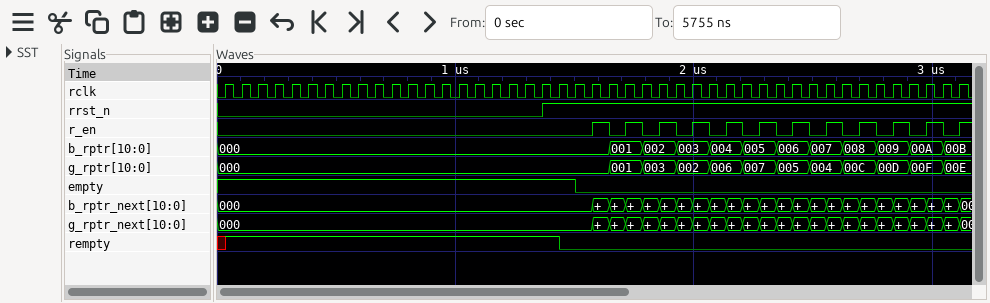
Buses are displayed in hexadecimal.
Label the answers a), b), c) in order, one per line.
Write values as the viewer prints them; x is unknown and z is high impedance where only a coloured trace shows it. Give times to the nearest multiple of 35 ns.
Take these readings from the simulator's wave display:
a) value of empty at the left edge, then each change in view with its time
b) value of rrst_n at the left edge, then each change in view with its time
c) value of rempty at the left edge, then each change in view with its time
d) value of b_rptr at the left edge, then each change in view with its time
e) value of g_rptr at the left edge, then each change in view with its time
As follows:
a) 1, 0 at 1505 ns
b) 0, 1 at 1365 ns
c) x, 1 at 35 ns, 0 at 1435 ns
d) 000, 001 at 1645 ns, 002 at 1785 ns, 003 at 1925 ns, 004 at 2065 ns, 005 at 2205 ns, 006 at 2345 ns, 007 at 2485 ns, 008 at 2625 ns, 009 at 2765 ns, 00A at 2905 ns, 00B at 3045 ns
e) 000, 001 at 1645 ns, 003 at 1785 ns, 002 at 1925 ns, 006 at 2065 ns, 007 at 2205 ns, 005 at 2345 ns, 004 at 2485 ns, 00C at 2625 ns, 00D at 2765 ns, 00F at 2905 ns, 00E at 3045 ns
